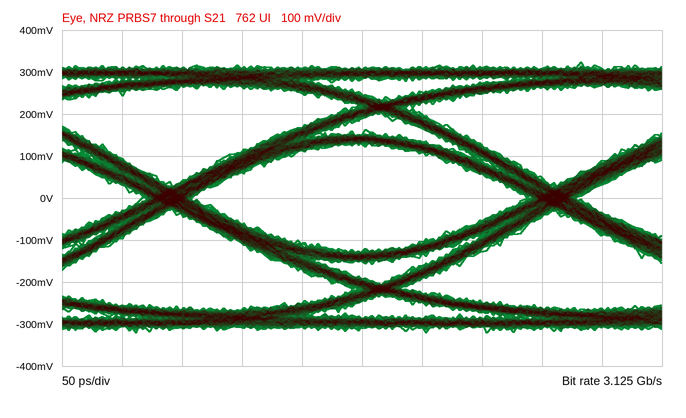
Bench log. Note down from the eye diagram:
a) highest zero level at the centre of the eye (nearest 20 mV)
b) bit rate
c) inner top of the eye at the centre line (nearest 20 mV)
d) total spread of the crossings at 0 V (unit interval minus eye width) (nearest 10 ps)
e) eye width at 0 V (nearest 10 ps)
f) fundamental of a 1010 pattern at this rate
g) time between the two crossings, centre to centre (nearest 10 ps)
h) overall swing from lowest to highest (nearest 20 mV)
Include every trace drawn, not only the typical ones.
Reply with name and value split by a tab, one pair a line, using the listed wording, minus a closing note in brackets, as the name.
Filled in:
highest zero level at the centre of the eye	-120 mV
bit rate	3.125 Gb/s
inner top of the eye at the centre line	120 mV
total spread of the crossings at 0 V (unit interval minus eye width)	40 ps
eye width at 0 V	280 ps
fundamental of a 1010 pattern at this rate	1.5625 GHz
time between the two crossings, centre to centre	320 ps
overall swing from lowest to highest	640 mV
